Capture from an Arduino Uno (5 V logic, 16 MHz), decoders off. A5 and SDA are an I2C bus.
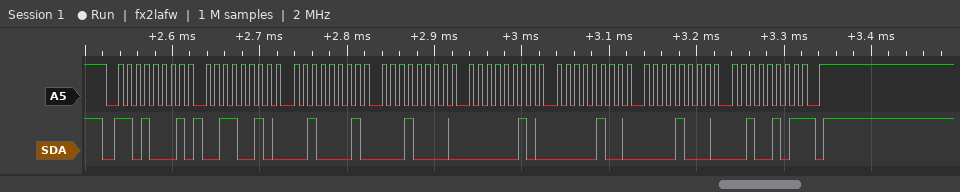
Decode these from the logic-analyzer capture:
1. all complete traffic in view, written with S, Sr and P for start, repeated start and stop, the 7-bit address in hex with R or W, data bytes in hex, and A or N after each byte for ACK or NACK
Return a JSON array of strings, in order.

["S 68R A 32 A 21 A 10 A 02 A 04 A 08 A 25 N P"]
